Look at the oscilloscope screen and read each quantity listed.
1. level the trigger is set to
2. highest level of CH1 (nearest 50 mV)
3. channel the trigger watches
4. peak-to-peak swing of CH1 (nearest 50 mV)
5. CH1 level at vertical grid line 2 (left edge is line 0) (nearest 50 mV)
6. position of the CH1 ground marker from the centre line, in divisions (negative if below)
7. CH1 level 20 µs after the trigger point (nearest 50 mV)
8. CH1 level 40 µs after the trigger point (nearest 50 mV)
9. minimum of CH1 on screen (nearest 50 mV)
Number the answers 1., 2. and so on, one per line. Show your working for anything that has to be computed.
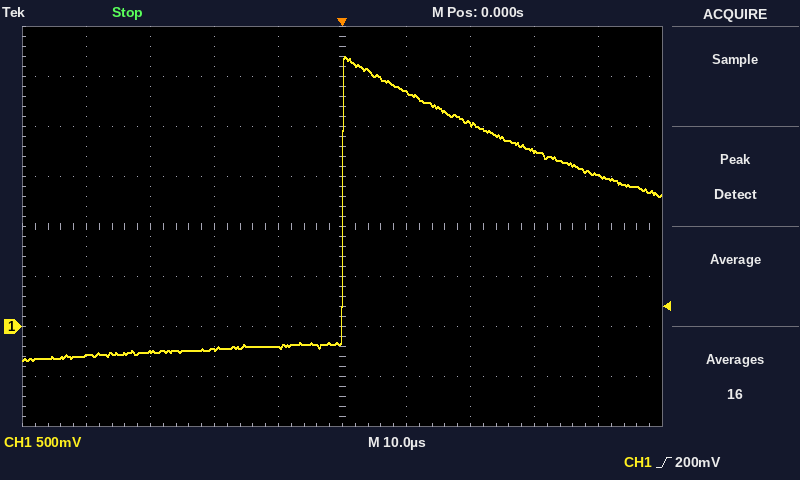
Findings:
1. 200 mV
2. 2.70 V
3. CH1
4. 2.70 V − (-350 mV) = 3.05 V
5. -250 mV
6. -2.0 div
7. 2.05 V
8. 1.50 V
9. -350 mV
